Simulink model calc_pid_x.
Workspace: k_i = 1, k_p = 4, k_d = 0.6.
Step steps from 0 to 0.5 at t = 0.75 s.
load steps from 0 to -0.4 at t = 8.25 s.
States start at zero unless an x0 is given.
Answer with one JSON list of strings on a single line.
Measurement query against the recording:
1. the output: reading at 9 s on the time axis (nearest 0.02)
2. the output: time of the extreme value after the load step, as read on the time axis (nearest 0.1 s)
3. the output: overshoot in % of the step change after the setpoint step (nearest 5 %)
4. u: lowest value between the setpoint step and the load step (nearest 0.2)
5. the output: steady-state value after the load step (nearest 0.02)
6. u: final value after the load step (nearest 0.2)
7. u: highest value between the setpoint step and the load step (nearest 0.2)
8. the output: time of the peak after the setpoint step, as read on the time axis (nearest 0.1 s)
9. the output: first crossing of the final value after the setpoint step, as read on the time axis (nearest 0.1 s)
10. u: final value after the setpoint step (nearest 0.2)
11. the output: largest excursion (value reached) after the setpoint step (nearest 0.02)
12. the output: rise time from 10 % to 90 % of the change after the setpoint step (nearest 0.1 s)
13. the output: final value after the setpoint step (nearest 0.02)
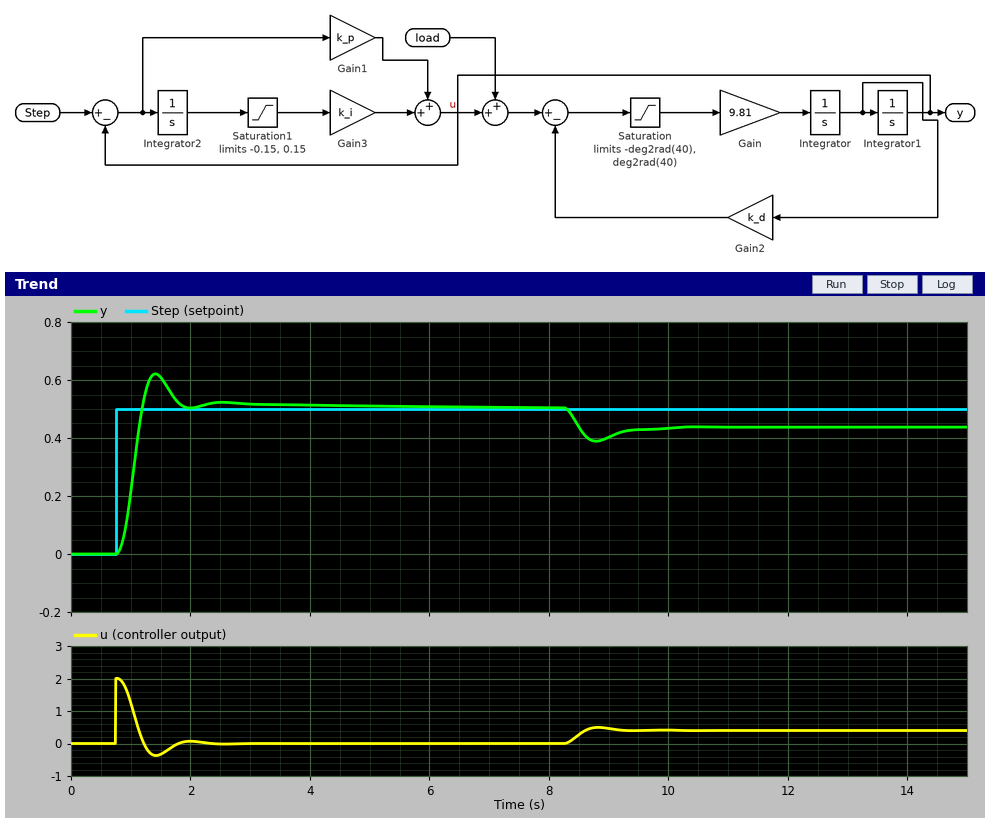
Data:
["0.40", "8.8 s", "25 %", "-0.4", "0.44", "0.4", "2.0", "1.4 s", "1.2 s", "0.0", "0.62", "0.3 s", "0.50"]
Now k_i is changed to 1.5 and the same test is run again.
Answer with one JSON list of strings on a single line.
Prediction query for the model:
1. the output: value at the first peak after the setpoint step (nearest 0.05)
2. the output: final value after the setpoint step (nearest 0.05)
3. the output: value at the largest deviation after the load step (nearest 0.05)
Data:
["0.65", "0.50", "0.40"]
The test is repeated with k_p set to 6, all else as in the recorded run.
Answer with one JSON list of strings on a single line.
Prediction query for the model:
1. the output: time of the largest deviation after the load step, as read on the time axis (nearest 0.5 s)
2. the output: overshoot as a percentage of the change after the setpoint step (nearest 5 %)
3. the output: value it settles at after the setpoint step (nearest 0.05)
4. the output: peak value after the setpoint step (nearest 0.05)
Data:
["8.5 s", "35 %", "0.50", "0.65"]
